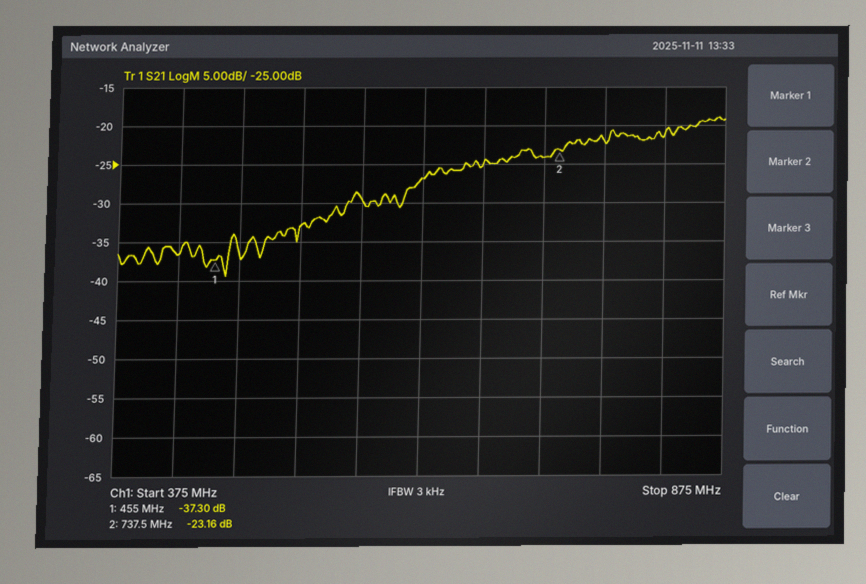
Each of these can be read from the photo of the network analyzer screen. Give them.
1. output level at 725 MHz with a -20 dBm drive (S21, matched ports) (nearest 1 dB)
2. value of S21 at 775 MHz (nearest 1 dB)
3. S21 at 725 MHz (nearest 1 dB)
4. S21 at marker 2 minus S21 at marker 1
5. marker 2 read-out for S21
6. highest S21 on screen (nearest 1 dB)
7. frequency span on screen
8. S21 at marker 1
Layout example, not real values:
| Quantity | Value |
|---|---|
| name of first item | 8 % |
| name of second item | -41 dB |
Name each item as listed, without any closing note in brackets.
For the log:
| Quantity | Value |
|---|---|
| output level at 725 MHz with a -20 dBm drive (S21, matched ports) | -44 dBm |
| value of S21 at 775 MHz | -22 dB |
| S21 at 725 MHz | -24 dB |
| S21 at marker 2 minus S21 at marker 1 | 14.14 dB |
| marker 2 read-out for S21 | -23.16 dB |
| highest S21 on screen | -19 dB |
| frequency span on screen | 500 MHz |
| S21 at marker 1 | -37.30 dB |
